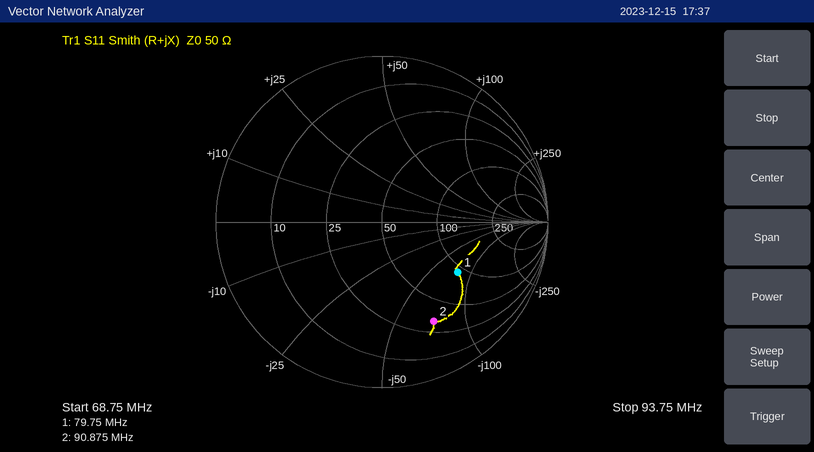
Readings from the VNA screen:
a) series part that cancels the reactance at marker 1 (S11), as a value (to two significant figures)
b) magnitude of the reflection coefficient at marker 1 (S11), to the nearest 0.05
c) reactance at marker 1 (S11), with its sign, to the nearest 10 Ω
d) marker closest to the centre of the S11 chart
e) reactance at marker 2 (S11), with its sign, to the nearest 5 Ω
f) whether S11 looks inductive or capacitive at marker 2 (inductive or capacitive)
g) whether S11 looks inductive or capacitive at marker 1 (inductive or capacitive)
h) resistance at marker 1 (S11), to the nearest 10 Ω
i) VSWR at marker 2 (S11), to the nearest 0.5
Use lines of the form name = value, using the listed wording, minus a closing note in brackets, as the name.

series part that cancels the reactance at marker 1 (S11), as a value = 160 nH
magnitude of the reflection coefficient at marker 1 (S11), to the nearest 0.05 = 0.55
reactance at marker 1 (S11), with its sign, to the nearest 10 Ω = -80 Ω
marker closest to the centre of the S11 chart = marker 1
reactance at marker 2 (S11), with its sign, to the nearest 5 Ω = -70 Ω
whether S11 looks inductive or capacitive at marker 2 = capacitive
whether S11 looks inductive or capacitive at marker 1 = capacitive
resistance at marker 1 (S11), to the nearest 10 Ω = 90 Ω
VSWR at marker 2 (S11), to the nearest 0.5 = 5.0
